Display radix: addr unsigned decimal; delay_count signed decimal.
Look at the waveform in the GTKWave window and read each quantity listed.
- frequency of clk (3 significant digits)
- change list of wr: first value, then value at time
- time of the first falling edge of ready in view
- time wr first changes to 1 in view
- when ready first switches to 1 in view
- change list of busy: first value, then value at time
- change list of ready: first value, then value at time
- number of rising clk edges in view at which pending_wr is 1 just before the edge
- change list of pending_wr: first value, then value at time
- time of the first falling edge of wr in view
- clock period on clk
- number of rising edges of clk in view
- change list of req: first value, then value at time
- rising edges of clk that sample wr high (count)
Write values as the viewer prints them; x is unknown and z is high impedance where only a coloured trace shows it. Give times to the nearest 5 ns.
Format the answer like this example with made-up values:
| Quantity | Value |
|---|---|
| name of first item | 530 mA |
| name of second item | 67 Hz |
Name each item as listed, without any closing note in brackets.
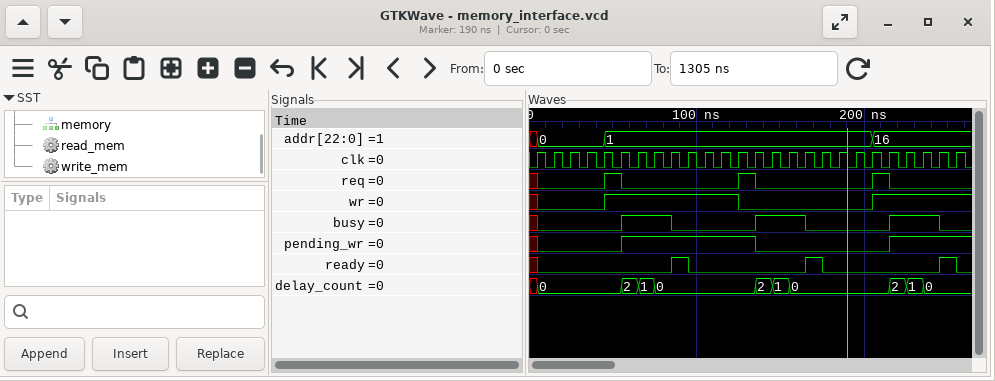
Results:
| Quantity | Value |
|---|---|
| frequency of clk | 100 MHz |
| change list of wr: first value, then value at time | x, 0 at 5 ns, 1 at 45 ns, 0 at 125 ns, 1 at 205 ns |
| time of the first falling edge of ready in view | 95 ns |
| time wr first changes to 1 in view | 45 ns |
| when ready first switches to 1 in view | 85 ns |
| change list of busy: first value, then value at time | x, 0 at 5 ns, 1 at 55 ns, 0 at 85 ns, 1 at 135 ns, 0 at 165 ns, 1 at 215 ns, 0 at 245 ns |
| change list of ready: first value, then value at time | x, 0 at 5 ns, 1 at 85 ns, 0 at 95 ns, 1 at 165 ns, 0 at 175 ns, 1 at 245 ns, 0 at 255 ns |
| number of rising clk edges in view at which pending_wr is 1 just before the edge | 12 |
| change list of pending_wr: first value, then value at time | x, 0 at 5 ns, 1 at 55 ns, 0 at 135 ns, 1 at 215 ns |
| time of the first falling edge of wr in view | 125 ns |
| clock period on clk | 10 ns |
| number of rising edges of clk in view | 26 |
| change list of req: first value, then value at time | x, 0 at 5 ns, 1 at 45 ns, 0 at 55 ns, 1 at 125 ns, 0 at 135 ns, 1 at 205 ns, 0 at 215 ns |
| rising edges of clk that sample wr high | 13 |
